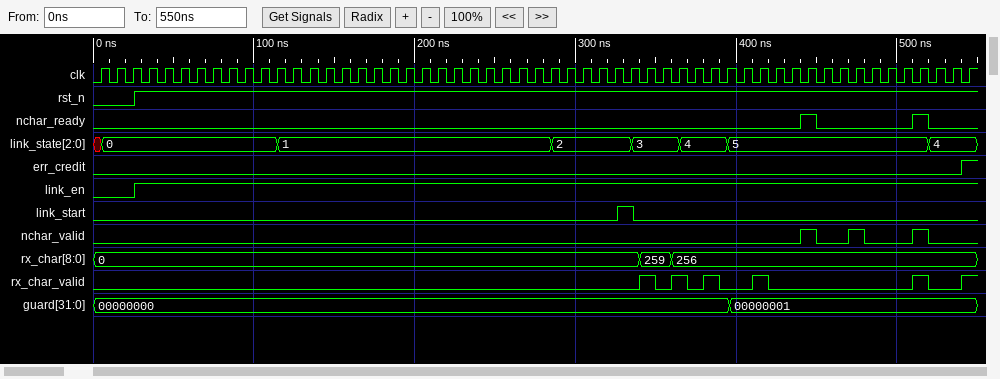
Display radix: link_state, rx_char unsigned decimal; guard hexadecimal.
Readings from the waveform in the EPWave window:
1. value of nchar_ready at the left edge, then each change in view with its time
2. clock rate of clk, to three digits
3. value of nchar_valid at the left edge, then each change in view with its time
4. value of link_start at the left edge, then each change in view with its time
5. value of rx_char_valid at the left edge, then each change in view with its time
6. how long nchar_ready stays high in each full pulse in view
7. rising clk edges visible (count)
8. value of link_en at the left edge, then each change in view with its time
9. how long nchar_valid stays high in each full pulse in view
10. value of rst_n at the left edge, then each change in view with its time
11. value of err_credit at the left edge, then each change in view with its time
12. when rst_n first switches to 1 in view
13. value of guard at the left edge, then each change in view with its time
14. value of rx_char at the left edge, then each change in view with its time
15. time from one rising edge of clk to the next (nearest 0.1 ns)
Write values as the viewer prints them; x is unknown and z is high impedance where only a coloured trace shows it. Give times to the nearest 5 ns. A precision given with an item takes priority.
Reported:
0, 1 at 440 ns, 0 at 450 ns, 1 at 510 ns, 0 at 520 ns
100 MHz
0, 1 at 440 ns, 0 at 450 ns, 1 at 470 ns, 0 at 480 ns, 1 at 510 ns, 0 at 520 ns
0, 1 at 325 ns, 0 at 335 ns
0, 1 at 340 ns, 0 at 350 ns, 1 at 360 ns, 0 at 370 ns, 1 at 380 ns, 0 at 390 ns, 1 at 410 ns, 0 at 420 ns, 1 at 510 ns, 0 at 520 ns, 1 at 540 ns
10 ns, 10 ns
55
0, 1 at 25 ns
10 ns, 10 ns, 10 ns
0, 1 at 25 ns
0, 1 at 540 ns
25 ns
00000000, 00000001 at 395 ns
0, 259 at 340 ns, 256 at 360 ns
10 ns
